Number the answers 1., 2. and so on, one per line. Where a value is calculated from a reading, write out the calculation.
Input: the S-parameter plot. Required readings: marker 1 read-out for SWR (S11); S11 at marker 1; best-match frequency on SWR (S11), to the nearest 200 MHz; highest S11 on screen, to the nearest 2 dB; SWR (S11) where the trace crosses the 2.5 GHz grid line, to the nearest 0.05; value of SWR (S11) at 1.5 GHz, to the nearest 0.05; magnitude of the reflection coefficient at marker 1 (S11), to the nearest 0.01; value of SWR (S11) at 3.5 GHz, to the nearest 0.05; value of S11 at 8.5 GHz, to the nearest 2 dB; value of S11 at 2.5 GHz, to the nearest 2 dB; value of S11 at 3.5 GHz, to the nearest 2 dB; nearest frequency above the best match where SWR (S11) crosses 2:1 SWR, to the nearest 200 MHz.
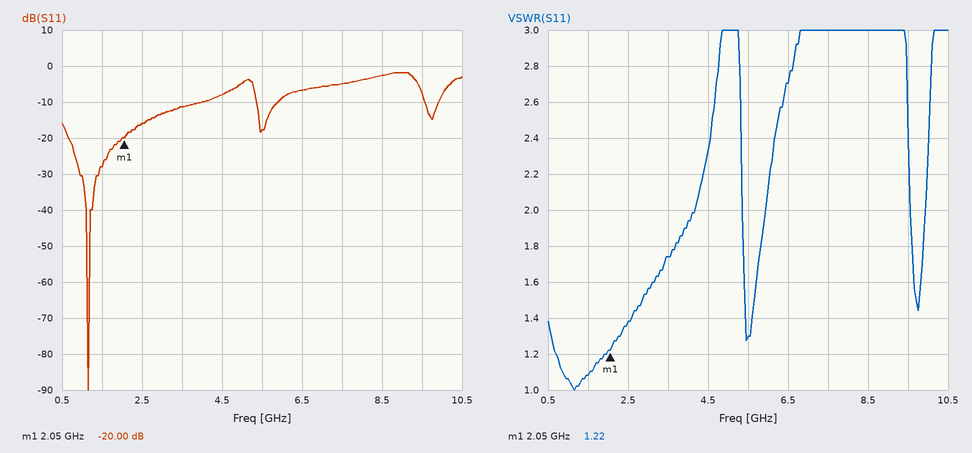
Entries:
1. 1.22
2. -20.00 dB
3. 1.2 GHz
4. -2 dB
5. 1.40
6. 1.10
7. 10^(-20/20) ≈ 0.10
8. 1.75
9. -2 dB
10. -16 dB
11. -12 dB
12. 4.2 GHz
